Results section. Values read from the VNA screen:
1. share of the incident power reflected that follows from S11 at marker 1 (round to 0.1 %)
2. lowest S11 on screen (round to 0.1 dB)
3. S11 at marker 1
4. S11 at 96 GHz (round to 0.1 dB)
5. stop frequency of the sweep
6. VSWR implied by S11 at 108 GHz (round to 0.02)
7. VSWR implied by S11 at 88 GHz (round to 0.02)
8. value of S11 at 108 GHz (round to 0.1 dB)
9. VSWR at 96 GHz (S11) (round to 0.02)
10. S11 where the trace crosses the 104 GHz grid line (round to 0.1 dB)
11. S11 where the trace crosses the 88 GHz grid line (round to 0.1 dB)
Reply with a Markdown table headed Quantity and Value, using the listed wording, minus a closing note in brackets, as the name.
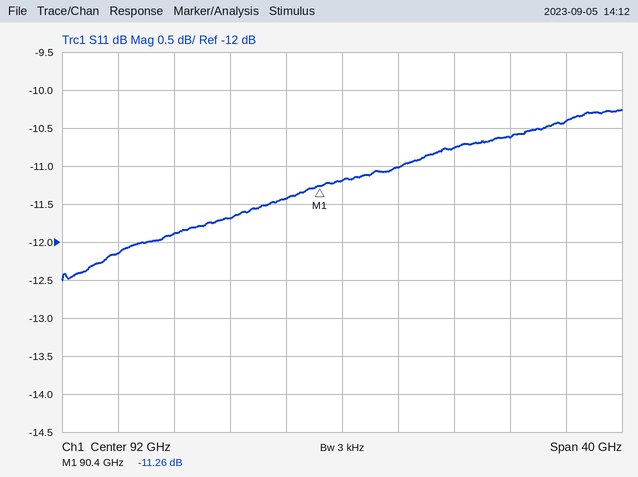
| Quantity | Value |
|---|---|
| share of the incident power reflected that follows from S11 at marker 1 | 7.5 % |
| lowest S11 on screen | -12.5 dB |
| S11 at marker 1 | -11.26 dB |
| S11 at 96 GHz | -11.0 dB |
| stop frequency of the sweep | 112 GHz |
| VSWR implied by S11 at 108 GHz | 1.86 |
| VSWR implied by S11 at 88 GHz | 1.74 |
| value of S11 at 108 GHz | -10.4 dB |
| VSWR at 96 GHz (S11) | 1.78 |
| S11 where the trace crosses the 104 GHz grid line | -10.6 dB |
| S11 where the trace crosses the 88 GHz grid line | -11.4 dB |
